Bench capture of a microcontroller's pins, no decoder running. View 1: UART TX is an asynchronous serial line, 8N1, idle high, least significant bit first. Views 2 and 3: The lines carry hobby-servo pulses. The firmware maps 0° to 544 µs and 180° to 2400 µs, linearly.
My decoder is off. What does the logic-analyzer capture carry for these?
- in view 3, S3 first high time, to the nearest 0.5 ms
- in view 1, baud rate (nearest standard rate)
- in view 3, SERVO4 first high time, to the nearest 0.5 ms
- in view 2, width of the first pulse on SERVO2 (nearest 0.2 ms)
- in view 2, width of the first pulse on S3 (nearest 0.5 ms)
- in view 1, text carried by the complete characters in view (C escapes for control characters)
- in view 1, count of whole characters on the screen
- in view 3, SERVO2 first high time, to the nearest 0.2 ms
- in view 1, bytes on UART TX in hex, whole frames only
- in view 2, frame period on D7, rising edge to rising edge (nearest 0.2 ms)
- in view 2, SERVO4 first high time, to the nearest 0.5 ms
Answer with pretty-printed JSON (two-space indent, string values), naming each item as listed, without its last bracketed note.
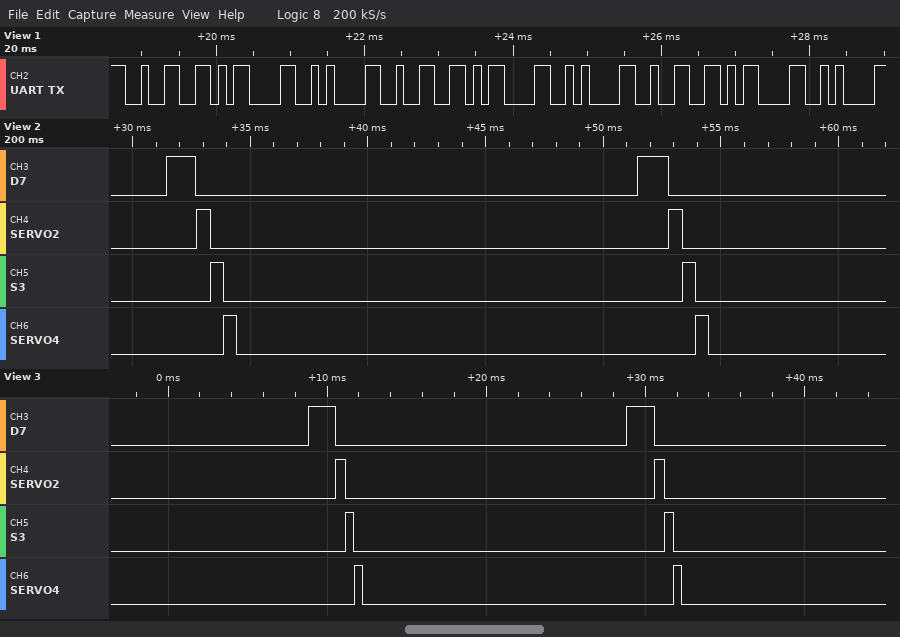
{
  "in view 3, S3 first high time, to the nearest 0.5 ms": "0.5 ms",
  "in view 1, baud rate": "9600 baud",
  "in view 3, SERVO4 first high time, to the nearest 0.5 ms": "0.5 ms",
  "in view 2, width of the first pulse on SERVO2": "0.6 ms",
  "in view 2, width of the first pulse on S3": "0.5 ms",
  "in view 1, text carried by the complete characters in view": "\"2\\r\\n2\\r\\n2\\r\\n\"",
  "in view 1, count of whole characters on the screen": "9",
  "in view 3, SERVO2 first high time, to the nearest 0.2 ms": "0.6 ms",
  "in view 1, bytes on UART TX in hex, whole frames only": "32 0D 0A 32 0D 0A 32 0D 0A",
  "in view 2, frame period on D7, rising edge to rising edge": "20.0 ms",
  "in view 2, SERVO4 first high time, to the nearest 0.5 ms": "0.5 ms"
}
